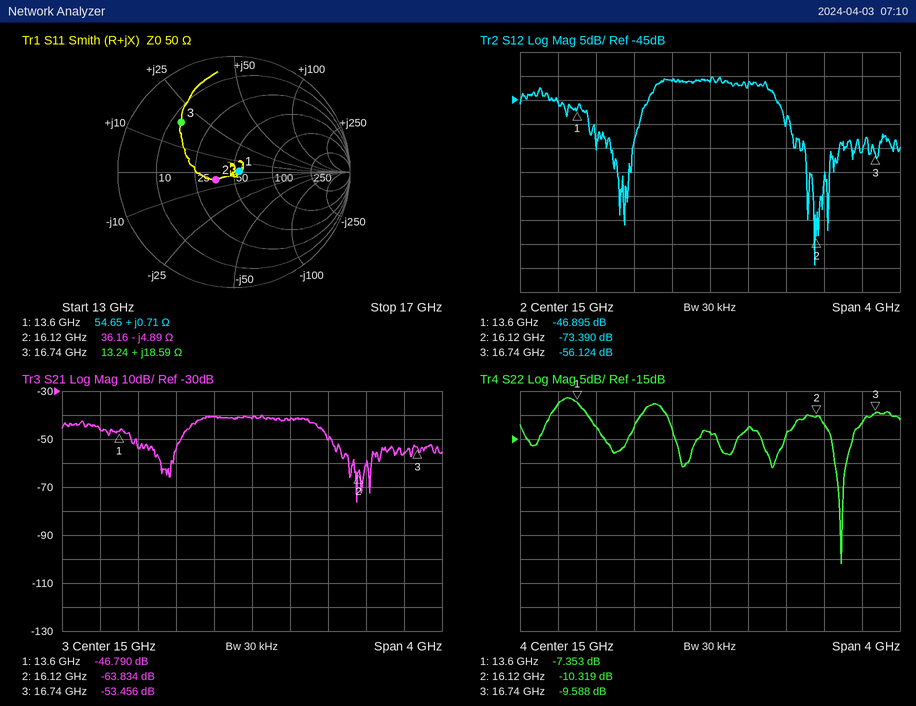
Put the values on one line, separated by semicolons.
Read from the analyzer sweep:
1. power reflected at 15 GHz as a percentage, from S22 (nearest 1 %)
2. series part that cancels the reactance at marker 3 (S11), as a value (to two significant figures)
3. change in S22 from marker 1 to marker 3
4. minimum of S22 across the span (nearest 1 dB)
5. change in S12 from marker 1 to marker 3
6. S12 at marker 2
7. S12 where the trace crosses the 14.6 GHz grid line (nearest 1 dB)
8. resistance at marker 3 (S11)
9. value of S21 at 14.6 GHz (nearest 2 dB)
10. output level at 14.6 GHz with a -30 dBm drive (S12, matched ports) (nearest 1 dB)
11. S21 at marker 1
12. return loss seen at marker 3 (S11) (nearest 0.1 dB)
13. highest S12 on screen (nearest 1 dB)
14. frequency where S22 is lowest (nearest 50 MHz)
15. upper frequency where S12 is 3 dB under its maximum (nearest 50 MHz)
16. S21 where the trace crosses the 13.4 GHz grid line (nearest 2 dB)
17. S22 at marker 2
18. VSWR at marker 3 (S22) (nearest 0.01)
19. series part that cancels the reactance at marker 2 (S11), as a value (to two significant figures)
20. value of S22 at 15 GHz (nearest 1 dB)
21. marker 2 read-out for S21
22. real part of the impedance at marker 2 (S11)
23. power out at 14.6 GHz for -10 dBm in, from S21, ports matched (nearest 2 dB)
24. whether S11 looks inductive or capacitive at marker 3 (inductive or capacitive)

4 %; 510 fF; -2.235 dB; -41 dB; -9.229 dB; -73.390 dB; -41 dB; 13.24 Ω; -40 dB; -71 dBm; -46.790 dB; 4.1 dB; -40 dB; 16.40 GHz; 15.65 GHz; -46 dB; -10.319 dB; 1.99; 48 pH; -14 dB; -63.834 dB; 36.16 Ω; -50 dBm; inductive
